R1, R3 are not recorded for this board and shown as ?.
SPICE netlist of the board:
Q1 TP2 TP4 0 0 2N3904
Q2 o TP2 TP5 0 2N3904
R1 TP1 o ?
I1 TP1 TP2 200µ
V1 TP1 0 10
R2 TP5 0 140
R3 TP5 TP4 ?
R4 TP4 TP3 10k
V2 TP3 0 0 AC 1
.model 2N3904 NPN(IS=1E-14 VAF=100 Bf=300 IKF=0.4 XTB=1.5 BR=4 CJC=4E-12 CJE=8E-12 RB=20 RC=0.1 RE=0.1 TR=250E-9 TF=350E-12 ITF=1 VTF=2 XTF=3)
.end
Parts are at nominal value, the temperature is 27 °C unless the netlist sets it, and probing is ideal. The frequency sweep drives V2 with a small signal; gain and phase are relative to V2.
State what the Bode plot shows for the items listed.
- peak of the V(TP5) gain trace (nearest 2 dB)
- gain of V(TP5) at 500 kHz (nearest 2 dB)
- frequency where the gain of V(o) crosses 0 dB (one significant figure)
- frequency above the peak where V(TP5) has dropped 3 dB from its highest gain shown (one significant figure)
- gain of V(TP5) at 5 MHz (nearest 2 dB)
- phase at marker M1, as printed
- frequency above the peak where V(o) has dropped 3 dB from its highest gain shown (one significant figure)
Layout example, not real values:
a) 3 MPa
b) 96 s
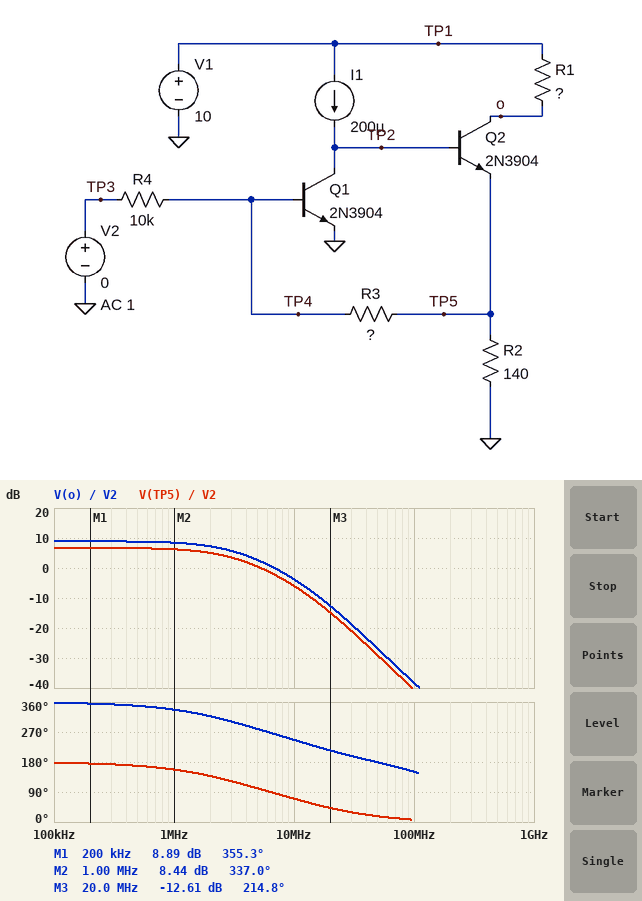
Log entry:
a) 6 dB
b) 6 dB
c) 7 MHz
d) 3 MHz
e) 0 dB
f) 355.3 deg
g) 3 MHz
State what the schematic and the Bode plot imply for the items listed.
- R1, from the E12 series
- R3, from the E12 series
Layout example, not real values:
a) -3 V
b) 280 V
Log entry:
a) 180 Ω
b) 22 kΩ
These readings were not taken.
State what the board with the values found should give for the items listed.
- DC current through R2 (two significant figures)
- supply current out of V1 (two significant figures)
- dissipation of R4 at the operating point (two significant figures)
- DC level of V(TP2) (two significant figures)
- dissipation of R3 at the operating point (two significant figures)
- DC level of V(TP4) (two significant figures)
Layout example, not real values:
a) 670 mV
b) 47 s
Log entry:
a) 14 mA
b) 14 mA
c) 37 µW
d) 2.7 V
e) 82 µW
f) 610 mV
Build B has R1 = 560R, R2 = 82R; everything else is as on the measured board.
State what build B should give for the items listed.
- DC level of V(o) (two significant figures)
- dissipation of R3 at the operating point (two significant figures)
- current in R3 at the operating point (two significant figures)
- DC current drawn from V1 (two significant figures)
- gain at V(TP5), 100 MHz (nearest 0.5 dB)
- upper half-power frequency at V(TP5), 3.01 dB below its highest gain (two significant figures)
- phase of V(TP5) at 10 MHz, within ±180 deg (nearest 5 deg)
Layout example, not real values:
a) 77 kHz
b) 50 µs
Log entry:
a) 1.4 V
b) 35 µW
c) 40 µA
d) 16 mA
e) -56.5 dB
f) 12 MHz
g) -5 deg
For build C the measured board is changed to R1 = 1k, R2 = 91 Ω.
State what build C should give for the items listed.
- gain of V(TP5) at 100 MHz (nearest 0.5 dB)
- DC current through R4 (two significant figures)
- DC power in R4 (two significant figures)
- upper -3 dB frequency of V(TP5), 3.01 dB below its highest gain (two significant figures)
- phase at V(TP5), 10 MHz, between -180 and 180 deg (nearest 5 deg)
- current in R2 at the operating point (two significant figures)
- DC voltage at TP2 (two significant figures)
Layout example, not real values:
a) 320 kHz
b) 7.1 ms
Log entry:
a) -54.0 dB
b) 26 µA
c) 6.9 µW
d) 260 MHz
e) -5 deg
f) 9.3 mA
g) 1.6 V
